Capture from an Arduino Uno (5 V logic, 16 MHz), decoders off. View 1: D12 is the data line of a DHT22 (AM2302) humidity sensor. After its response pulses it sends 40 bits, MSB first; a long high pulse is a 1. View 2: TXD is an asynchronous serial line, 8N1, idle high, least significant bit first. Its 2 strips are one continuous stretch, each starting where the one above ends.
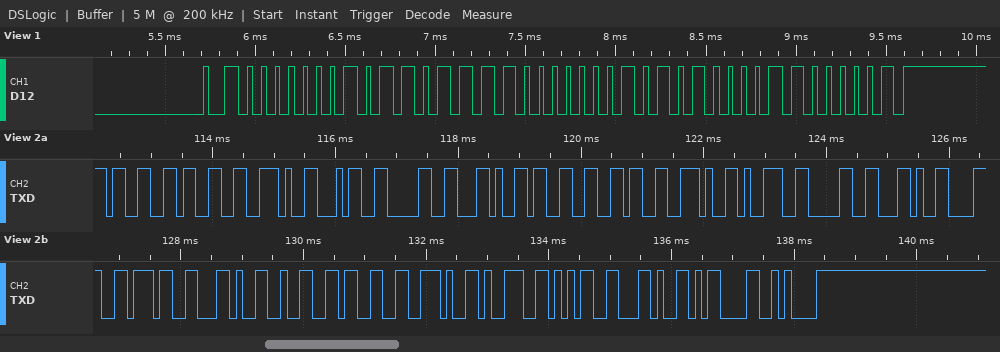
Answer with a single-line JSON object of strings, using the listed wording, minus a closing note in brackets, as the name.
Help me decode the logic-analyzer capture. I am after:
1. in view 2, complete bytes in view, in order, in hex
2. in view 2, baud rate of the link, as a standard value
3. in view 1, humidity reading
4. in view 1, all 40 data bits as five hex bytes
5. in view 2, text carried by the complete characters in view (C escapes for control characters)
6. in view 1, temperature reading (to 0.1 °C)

{"in view 2, complete bytes in view, in order, in hex": "0x33 0x33 0x2E 0x34 0x30 0x2C 0x33 0x36 0x2E 0x39 0x30 0x2C 0x38 0x37 0x2C 0x32 0x33 0x2E 0x39 0x35 0x2C 0x0D 0x0A", "in view 2, baud rate of the link, as a standard value": "9600 baud", "in view 1, humidity reading": "36.7 %", "in view 1, all 40 data bits as five hex bytes": "01 6F 01 50 C1", "in view 2, text carried by the complete characters in view": "\"33.40,36.90,87,23.95,\\r\\n\"", "in view 1, temperature reading": "33.6 °C"}
